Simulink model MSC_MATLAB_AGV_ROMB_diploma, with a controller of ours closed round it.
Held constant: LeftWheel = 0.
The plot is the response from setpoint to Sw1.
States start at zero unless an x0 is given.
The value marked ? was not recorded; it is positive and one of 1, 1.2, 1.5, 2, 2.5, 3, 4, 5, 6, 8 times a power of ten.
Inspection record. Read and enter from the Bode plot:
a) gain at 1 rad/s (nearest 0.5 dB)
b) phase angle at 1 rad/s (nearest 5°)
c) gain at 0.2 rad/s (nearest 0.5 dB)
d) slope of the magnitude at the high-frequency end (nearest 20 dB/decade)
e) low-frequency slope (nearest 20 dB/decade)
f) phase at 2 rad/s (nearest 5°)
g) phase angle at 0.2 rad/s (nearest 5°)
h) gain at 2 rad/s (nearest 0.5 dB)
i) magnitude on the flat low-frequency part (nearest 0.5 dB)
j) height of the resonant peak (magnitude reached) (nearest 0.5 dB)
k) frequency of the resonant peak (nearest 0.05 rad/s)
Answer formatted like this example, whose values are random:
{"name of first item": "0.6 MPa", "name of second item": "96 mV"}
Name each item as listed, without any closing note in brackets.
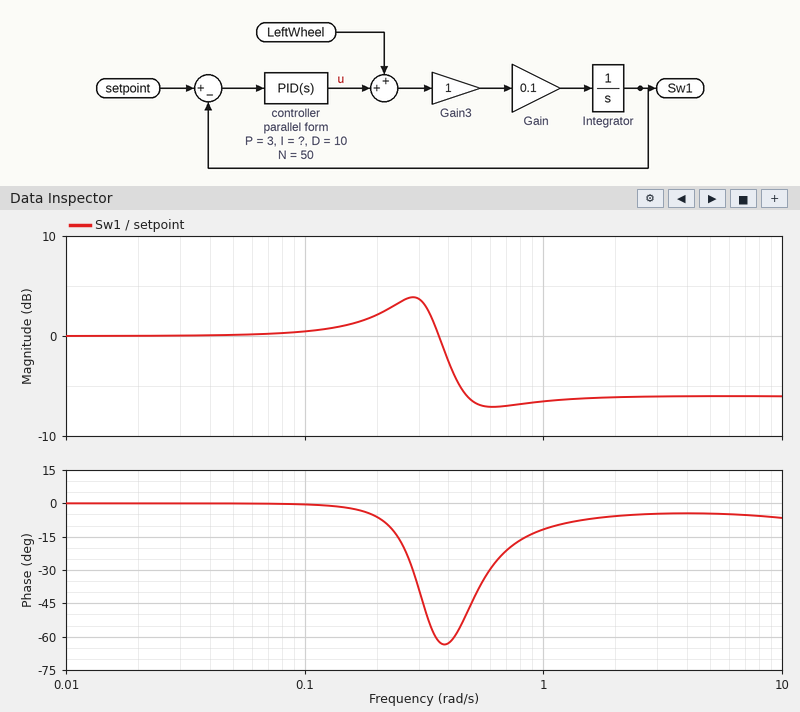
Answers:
{"gain at 1 rad/s": "-6.5 dB", "phase angle at 1 rad/s": "-10°", "gain at 0.2 rad/s": "2.0 dB", "slope of the magnitude at the high-frequency end": "0 dB/decade", "low-frequency slope": "0 dB/decade", "phase at 2 rad/s": "-5°", "phase angle at 0.2 rad/s": "-5°", "gain at 2 rad/s": "-6.0 dB", "magnitude on the flat low-frequency part": "0.0 dB", "height of the resonant peak (magnitude reached)": "4.0 dB", "frequency of the resonant peak": "0.30 rad/s"}
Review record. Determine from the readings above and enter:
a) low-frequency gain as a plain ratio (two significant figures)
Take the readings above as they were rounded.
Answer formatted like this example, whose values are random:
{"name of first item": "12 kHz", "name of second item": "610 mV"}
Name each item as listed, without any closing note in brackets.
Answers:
{"low-frequency gain as a plain ratio": "1.0"}
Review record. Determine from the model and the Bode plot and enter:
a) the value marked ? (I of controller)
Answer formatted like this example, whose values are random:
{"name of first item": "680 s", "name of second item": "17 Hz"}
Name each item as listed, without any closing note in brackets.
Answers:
{"the value marked ?": "2"}
